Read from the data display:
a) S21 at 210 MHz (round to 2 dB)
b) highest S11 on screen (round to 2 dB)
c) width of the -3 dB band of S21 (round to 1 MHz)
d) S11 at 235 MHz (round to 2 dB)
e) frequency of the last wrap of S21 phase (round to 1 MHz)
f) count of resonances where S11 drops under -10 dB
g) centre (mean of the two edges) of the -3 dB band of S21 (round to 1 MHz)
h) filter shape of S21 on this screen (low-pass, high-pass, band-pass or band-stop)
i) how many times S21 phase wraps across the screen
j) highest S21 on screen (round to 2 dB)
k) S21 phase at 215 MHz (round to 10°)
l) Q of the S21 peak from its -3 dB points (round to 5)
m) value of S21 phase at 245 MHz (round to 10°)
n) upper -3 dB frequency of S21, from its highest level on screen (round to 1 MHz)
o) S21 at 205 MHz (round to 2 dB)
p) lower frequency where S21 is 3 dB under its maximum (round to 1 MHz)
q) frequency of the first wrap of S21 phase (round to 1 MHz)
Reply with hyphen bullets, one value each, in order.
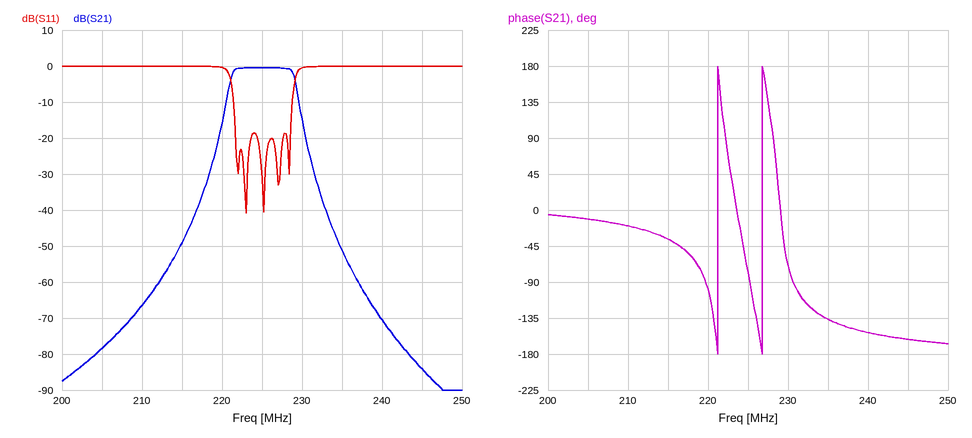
- -66 dB
- 0 dB
- 8 MHz
- 0 dB
- 227 MHz
- 5
- 225 MHz
- band-pass
- 2
- 0 dB
- -40°
- 30
- -160°
- 229 MHz
- -78 dB
- 221 MHz
- 221 MHz
